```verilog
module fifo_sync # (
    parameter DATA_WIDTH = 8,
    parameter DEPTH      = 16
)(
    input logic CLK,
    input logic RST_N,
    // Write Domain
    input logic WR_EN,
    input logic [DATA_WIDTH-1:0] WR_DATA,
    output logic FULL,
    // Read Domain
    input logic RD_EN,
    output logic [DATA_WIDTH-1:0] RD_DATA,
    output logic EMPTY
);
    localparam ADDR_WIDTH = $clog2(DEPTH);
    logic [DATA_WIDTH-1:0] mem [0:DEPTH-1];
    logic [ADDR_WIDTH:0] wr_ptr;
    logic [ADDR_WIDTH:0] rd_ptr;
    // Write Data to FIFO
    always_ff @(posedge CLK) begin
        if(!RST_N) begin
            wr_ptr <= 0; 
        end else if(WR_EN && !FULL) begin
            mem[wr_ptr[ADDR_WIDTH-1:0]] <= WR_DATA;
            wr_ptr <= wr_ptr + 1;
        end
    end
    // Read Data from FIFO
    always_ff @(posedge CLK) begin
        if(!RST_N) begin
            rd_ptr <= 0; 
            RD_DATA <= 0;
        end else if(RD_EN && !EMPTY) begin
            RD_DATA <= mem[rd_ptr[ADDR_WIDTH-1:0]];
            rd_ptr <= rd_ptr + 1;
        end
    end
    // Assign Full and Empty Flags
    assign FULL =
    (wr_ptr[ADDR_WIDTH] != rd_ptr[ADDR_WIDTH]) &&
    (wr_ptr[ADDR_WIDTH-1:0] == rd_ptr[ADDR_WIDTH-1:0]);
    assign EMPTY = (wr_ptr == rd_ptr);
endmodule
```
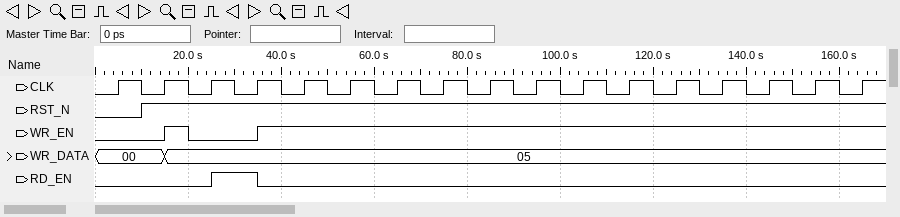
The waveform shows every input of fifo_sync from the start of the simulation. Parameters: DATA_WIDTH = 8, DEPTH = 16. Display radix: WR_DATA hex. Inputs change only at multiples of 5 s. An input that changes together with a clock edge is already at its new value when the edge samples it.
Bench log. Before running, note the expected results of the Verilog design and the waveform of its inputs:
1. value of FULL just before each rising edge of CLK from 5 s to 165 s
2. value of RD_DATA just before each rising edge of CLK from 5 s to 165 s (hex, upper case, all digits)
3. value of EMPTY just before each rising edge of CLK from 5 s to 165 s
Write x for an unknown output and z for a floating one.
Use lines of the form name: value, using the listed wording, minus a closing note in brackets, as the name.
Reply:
value of FULL just before each rising edge of CLK from 5 s to 165 s: x 0 0 0 0 0 0 0 0 0 0 0 0 0 0 0 0
value of RD_DATA just before each rising edge of CLK from 5 s to 165 s: x, 00, 00, 05, 05, 05, 05, 05, 05, 05, 05, 05, 05, 05, 05, 05, 05
value of EMPTY just before each rising edge of CLK from 5 s to 165 s: x 1 0 1 0 0 0 0 0 0 0 0 0 0 0 0 0
